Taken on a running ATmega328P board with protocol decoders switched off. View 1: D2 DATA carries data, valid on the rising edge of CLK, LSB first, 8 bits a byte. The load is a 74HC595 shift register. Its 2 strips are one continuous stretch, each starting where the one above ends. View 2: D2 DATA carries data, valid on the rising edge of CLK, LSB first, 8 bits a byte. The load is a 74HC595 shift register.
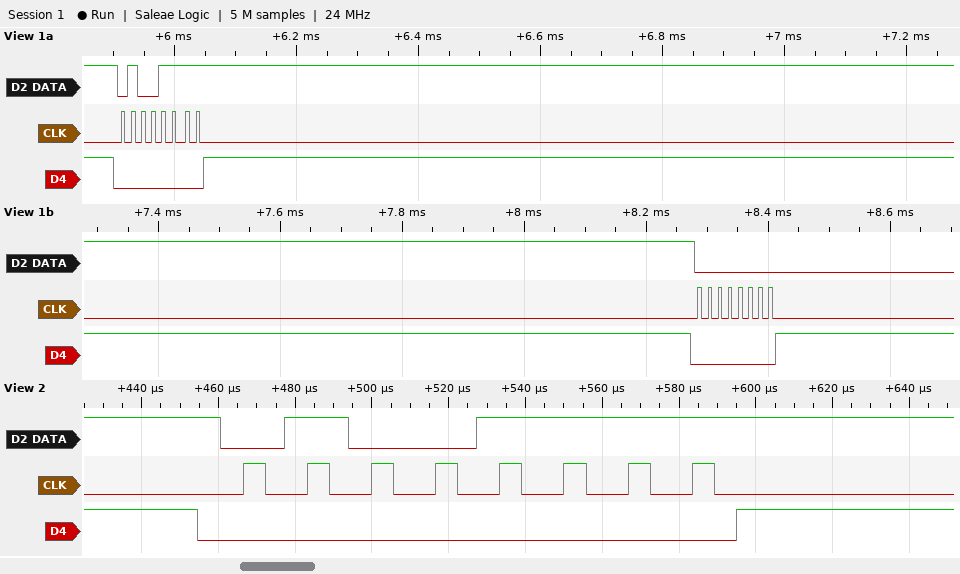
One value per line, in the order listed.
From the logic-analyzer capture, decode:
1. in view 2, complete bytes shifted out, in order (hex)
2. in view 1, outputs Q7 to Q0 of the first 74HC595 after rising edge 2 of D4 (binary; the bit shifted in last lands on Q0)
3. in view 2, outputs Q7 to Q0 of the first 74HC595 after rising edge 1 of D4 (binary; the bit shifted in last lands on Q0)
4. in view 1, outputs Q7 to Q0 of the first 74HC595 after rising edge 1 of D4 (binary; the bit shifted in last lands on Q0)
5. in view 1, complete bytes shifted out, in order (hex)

0xF2
00000000
01001111
01001111
F2 00
